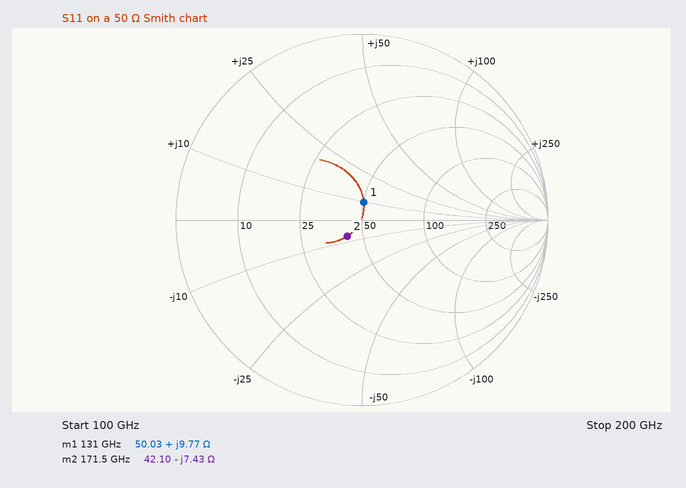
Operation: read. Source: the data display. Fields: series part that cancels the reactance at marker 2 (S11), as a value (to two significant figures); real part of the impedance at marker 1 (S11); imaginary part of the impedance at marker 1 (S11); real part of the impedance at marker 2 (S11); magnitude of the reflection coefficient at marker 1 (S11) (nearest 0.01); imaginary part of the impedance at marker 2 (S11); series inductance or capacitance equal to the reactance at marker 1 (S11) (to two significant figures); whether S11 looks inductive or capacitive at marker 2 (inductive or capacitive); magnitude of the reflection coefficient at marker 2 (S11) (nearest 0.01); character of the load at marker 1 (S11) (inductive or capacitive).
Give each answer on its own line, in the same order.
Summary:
6.9 pH
50.03 Ω
+9.77 Ω
42.10 Ω
0.10
-7.43 Ω
12 pH
capacitive
0.12
inductive
